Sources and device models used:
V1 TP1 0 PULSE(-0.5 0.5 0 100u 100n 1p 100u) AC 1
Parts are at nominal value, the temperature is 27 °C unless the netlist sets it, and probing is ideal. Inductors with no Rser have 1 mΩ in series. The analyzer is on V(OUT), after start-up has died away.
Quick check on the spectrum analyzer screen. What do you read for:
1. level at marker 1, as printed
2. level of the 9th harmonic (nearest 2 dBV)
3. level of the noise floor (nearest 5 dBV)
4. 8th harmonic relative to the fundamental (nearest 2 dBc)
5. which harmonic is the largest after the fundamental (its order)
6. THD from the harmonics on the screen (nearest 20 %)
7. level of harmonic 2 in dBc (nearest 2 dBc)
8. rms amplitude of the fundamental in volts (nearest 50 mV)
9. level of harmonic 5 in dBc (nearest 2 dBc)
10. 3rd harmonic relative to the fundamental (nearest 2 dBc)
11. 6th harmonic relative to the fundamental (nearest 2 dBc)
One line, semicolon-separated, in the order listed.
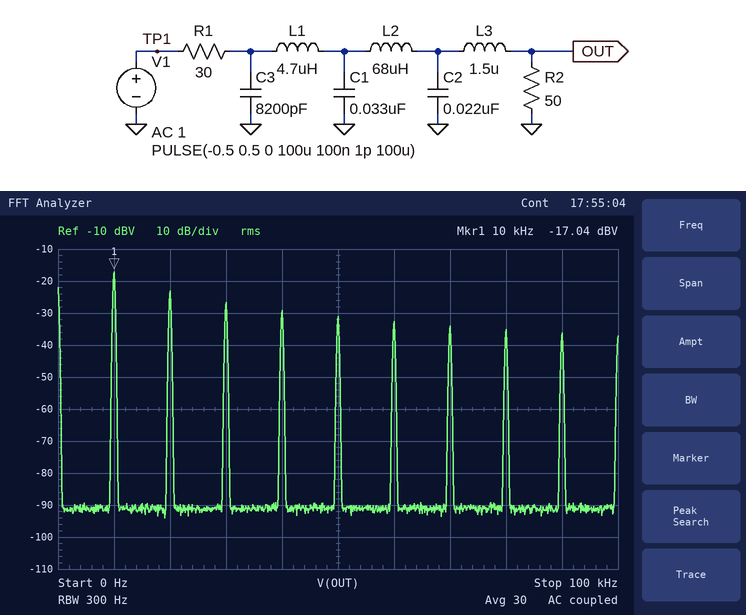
-17.04 dBV; -36 dBV; -90 dBV; -18 dBc; 2; 80 %; -6 dBc; 150 mV; -14 dBc; -10 dBc; -16 dBc
